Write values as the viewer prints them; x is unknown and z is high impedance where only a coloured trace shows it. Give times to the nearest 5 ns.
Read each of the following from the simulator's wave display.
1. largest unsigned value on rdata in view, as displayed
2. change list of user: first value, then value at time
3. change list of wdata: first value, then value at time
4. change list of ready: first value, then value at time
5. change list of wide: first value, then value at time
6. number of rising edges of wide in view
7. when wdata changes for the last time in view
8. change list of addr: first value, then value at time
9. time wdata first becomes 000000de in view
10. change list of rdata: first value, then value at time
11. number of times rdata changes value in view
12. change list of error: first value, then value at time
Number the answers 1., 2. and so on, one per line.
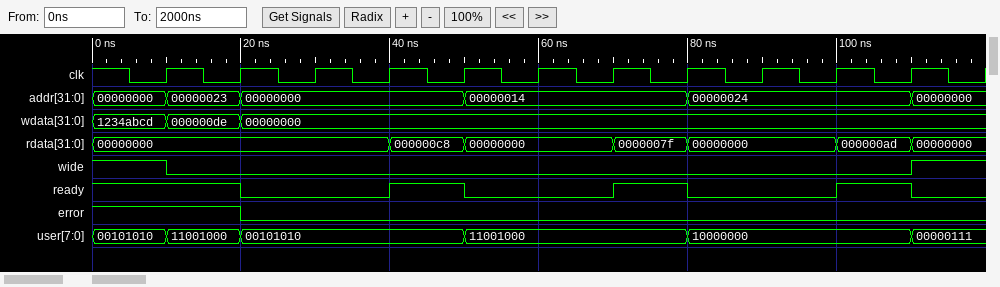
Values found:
1. 000000c8
2. 00101010, 11001000 at 10 ns, 00101010 at 20 ns, 11001000 at 50 ns, 10000000 at 80 ns, 00000111 at 110 ns
3. 1234abcd, 000000de at 10 ns, 00000000 at 20 ns
4. 1, 0 at 20 ns, 1 at 40 ns, 0 at 50 ns, 1 at 70 ns, 0 at 80 ns, 1 at 100 ns, 0 at 110 ns
5. 1, 0 at 10 ns, 1 at 110 ns
6. 1
7. 20 ns
8. 00000000, 00000023 at 10 ns, 00000000 at 20 ns, 00000014 at 50 ns, 00000024 at 80 ns, 00000000 at 110 ns
9. 10 ns
10. 00000000, 000000c8 at 40 ns, 00000000 at 50 ns, 0000007f at 70 ns, 00000000 at 80 ns, 000000ad at 100 ns, 00000000 at 110 ns
11. 6
12. 1, 0 at 20 ns
